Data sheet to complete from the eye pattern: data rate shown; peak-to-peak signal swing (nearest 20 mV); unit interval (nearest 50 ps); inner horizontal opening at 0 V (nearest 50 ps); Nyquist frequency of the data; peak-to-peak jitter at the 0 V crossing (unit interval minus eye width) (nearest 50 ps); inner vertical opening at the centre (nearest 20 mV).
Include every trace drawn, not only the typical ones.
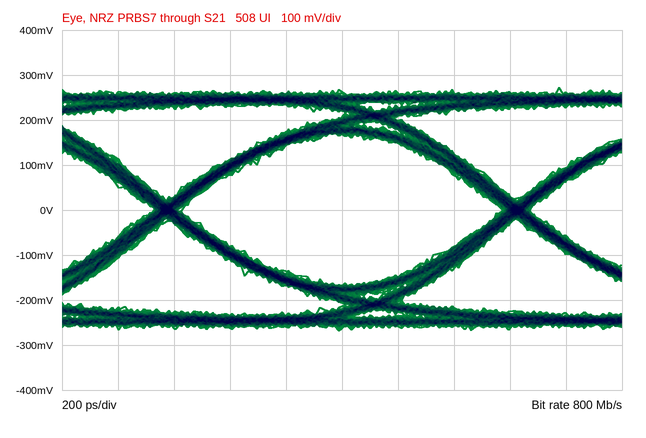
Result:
800 Mb/s
540 mV
1.25 ns
1.15 ns
400 MHz
100 ps
340 mV
